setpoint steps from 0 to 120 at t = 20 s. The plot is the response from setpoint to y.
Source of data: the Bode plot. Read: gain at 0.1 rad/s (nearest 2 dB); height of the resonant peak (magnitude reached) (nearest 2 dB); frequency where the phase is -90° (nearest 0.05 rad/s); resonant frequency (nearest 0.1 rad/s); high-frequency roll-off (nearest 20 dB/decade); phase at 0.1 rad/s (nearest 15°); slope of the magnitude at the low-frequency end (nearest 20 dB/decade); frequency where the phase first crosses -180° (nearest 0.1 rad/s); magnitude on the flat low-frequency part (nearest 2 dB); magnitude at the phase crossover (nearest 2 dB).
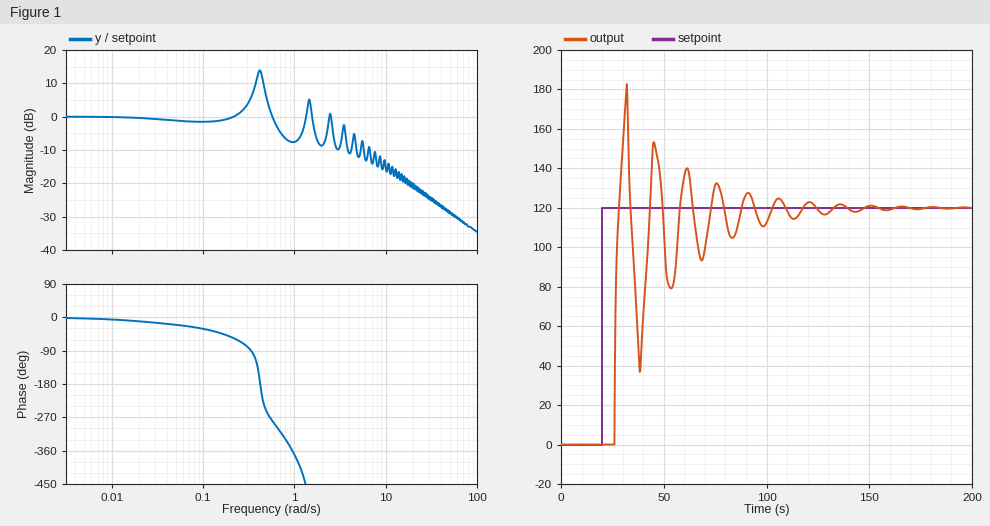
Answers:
-2 dB
14 dB
0.35 rad/s
0.4 rad/s
-20 dB/decade
-30°
0 dB/decade
0.4 rad/s
0 dB
14 dB
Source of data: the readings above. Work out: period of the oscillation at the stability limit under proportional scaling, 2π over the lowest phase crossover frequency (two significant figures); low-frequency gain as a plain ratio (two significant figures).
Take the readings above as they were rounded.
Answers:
16 s
1.0
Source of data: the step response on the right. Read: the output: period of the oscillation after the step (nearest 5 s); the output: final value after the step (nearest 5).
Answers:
15 s
120
